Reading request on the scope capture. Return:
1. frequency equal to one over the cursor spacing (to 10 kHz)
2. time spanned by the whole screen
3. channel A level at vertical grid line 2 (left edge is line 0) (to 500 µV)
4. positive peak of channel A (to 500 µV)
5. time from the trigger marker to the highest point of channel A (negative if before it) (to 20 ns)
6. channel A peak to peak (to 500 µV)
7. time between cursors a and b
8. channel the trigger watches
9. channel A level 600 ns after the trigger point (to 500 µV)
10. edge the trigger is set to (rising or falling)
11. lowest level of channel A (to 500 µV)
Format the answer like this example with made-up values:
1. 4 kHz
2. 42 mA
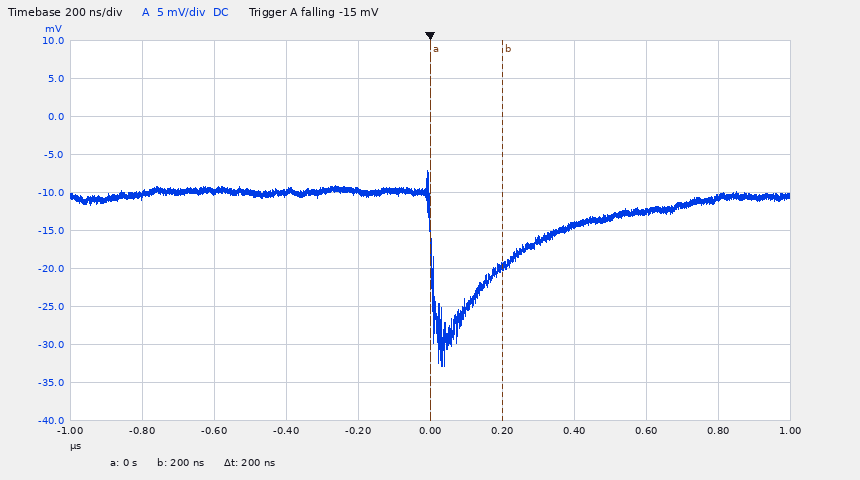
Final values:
1. 5.00 MHz
2. 2 µs
3. -10.0 mV
4. -7.0 mV
5. 0 ns
6. 26.0 mV
7. 200 ns
8. channel A
9. -12.5 mV
10. falling
11. -33.0 mV
